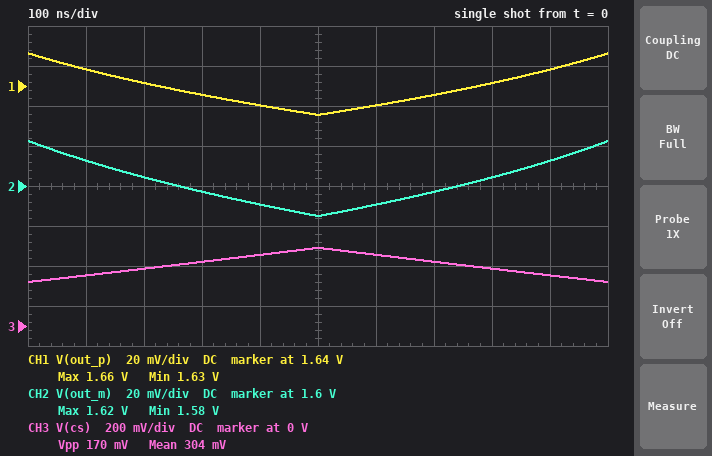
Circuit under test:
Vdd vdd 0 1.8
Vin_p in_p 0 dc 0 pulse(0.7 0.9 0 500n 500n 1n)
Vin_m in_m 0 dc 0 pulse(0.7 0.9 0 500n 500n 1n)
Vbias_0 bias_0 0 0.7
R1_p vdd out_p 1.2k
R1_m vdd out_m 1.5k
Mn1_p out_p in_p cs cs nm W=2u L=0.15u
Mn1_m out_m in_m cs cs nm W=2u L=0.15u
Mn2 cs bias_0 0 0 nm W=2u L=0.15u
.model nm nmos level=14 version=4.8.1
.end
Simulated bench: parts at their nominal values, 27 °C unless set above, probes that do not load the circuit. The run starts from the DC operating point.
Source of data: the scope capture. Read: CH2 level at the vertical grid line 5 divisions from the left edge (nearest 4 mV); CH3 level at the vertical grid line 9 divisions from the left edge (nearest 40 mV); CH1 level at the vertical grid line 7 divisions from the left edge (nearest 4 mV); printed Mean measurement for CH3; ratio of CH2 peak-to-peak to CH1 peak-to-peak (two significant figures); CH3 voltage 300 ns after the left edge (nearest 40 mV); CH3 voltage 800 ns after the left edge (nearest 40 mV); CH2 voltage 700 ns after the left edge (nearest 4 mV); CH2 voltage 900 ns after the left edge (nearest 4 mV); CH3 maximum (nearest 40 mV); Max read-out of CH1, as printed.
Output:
1.584 V
240 mV
1.636 V
304 mV
1.2
320 mV
280 mV
1.596 V
1.612 V
400 mV
1.66 V
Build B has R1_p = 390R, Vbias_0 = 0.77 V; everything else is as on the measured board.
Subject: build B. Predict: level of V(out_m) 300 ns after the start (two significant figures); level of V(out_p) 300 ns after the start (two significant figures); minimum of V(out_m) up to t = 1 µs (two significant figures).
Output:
1.6 V
1.7 V
1.5 V
